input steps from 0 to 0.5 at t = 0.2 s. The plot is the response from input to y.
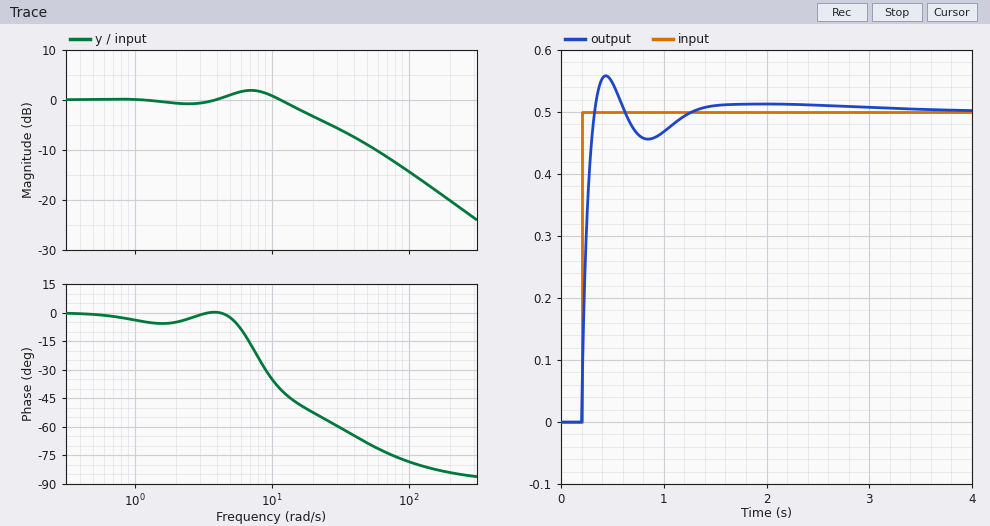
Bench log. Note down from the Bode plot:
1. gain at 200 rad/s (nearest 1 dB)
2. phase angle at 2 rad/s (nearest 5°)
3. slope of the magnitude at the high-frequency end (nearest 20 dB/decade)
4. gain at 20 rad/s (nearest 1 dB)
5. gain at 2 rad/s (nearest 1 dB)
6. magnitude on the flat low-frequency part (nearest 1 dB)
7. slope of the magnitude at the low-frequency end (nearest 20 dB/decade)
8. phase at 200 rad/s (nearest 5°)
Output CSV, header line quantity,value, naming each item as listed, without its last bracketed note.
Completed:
quantity,value
gain at 200 rad/s,-20 dB
phase angle at 2 rad/s,-5°
slope of the magnitude at the high-frequency end,-20 dB/decade
gain at 20 rad/s,-3 dB
gain at 2 rad/s,-1 dB
magnitude on the flat low-frequency part,0 dB
slope of the magnitude at the low-frequency end,0 dB/decade
phase at 200 rad/s,-85°
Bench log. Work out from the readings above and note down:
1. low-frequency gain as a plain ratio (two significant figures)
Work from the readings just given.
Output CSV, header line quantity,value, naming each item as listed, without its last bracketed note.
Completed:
quantity,value
low-frequency gain as a plain ratio,1.0
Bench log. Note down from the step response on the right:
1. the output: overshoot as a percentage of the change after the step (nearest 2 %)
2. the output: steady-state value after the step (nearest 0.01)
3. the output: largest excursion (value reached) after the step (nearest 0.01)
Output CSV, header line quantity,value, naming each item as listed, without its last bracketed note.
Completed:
quantity,value
the output: overshoot as a percentage of the change after the step,12 %
the output: steady-state value after the step,0.50
the output: largest excursion (value reached) after the step,0.56
